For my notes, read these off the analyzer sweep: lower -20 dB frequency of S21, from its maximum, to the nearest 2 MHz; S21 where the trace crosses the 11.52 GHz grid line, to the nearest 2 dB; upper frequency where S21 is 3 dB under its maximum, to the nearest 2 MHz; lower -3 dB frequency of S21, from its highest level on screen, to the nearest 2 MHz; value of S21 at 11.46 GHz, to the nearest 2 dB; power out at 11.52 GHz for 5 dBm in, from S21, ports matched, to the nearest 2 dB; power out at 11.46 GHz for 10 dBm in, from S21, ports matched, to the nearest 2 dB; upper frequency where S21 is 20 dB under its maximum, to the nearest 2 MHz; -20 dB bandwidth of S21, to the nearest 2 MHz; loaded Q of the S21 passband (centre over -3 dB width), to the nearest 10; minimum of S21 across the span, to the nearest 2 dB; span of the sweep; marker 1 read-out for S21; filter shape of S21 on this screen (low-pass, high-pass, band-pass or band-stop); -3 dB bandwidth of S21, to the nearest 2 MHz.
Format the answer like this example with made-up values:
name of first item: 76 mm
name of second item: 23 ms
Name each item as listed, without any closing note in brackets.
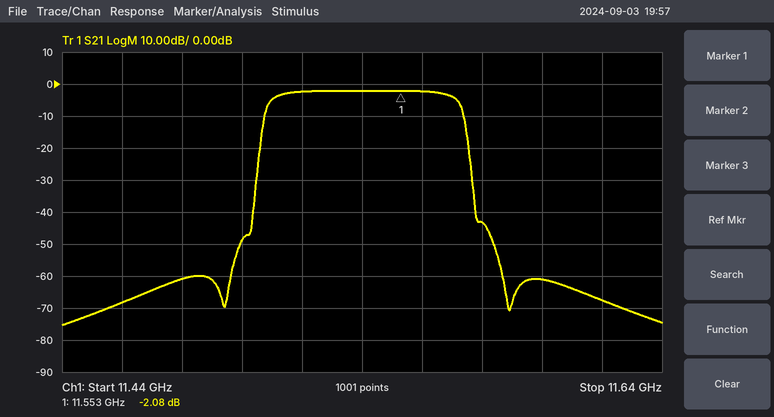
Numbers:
lower -20 dB frequency of S21, from its maximum, to the nearest 2 MHz: 11.506 GHz
S21 where the trace crosses the 11.52 GHz grid line, to the nearest 2 dB: -2 dB
upper frequency where S21 is 3 dB under its maximum, to the nearest 2 MHz: 11.572 GHz
lower -3 dB frequency of S21, from its highest level on screen, to the nearest 2 MHz: 11.510 GHz
value of S21 at 11.46 GHz, to the nearest 2 dB: -68 dB
power out at 11.52 GHz for 5 dBm in, from S21, ports matched, to the nearest 2 dB: 2 dBm
power out at 11.46 GHz for 10 dBm in, from S21, ports matched, to the nearest 2 dB: -58 dBm
upper frequency where S21 is 20 dB under its maximum, to the nearest 2 MHz: 11.576 GHz
-20 dB bandwidth of S21, to the nearest 2 MHz: 70 MHz
loaded Q of the S21 passband (centre over -3 dB width), to the nearest 10: 190
minimum of S21 across the span, to the nearest 2 dB: -76 dB
span of the sweep: 200 MHz
marker 1 read-out for S21: -2.08 dB
filter shape of S21 on this screen: band-pass
-3 dB bandwidth of S21, to the nearest 2 MHz: 62 MHz
